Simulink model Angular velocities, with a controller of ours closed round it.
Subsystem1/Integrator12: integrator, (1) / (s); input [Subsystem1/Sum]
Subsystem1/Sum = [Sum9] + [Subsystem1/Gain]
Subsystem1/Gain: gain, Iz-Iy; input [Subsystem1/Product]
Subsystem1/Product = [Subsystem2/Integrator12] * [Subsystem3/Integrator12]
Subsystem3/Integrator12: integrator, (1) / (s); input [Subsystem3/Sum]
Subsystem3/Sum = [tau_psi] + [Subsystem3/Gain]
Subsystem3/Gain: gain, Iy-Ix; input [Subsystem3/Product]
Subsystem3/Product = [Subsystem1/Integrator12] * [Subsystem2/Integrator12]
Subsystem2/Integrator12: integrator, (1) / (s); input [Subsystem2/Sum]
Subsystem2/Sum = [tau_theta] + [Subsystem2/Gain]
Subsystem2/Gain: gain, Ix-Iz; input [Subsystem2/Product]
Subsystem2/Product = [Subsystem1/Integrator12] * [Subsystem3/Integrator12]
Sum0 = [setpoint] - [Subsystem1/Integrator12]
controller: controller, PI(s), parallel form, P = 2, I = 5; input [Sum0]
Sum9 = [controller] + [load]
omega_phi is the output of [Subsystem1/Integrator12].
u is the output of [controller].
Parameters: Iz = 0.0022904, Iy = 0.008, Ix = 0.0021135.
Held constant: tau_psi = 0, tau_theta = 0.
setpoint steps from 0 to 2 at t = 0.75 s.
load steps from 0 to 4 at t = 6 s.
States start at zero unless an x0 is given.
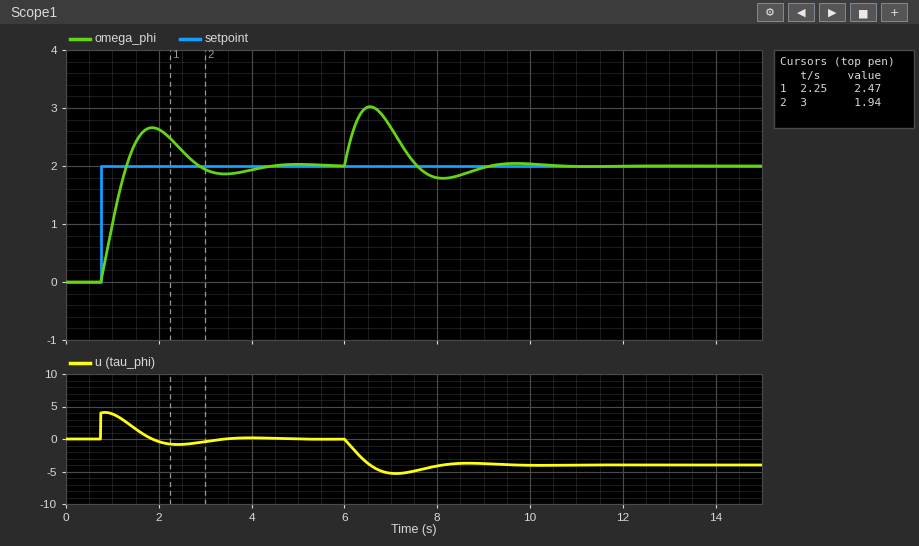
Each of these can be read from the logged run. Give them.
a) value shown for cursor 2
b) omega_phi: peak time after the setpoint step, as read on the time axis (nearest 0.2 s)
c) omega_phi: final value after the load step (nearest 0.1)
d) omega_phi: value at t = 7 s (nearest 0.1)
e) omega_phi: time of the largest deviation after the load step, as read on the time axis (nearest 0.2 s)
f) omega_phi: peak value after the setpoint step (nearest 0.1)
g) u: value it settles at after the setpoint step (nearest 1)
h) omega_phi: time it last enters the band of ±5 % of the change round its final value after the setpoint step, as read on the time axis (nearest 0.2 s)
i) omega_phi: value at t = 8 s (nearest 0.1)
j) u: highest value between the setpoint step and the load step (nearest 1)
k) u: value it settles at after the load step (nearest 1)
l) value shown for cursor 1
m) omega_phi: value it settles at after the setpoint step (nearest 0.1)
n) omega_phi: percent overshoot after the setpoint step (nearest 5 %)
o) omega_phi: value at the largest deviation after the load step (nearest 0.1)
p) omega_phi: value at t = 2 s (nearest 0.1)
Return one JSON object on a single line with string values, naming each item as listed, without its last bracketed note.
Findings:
{"value shown for cursor 2": "1.94", "omega_phi: peak time after the setpoint step, as read on the time axis": "1.8 s", "omega_phi: final value after the load step": "2.0", "omega_phi: value at t = 7 s": "2.7", "omega_phi: time of the largest deviation after the load step, as read on the time axis": "6.6 s", "omega_phi: peak value after the setpoint step": "2.7", "u: value it settles at after the setpoint step": "0", "omega_phi: time it last enters the band of ±5 % of the change round its final value after the setpoint step, as read on the time axis": "3.8 s", "omega_phi: value at t = 8 s": "1.8", "u: highest value between the setpoint step and the load step": "4", "u: value it settles at after the load step": "-4", "value shown for cursor 1": "2.47", "omega_phi: value it settles at after the setpoint step": "2.0", "omega_phi: percent overshoot after the setpoint step": "35 %", "omega_phi: value at the largest deviation after the load step": "3.0", "omega_phi: value at t = 2 s": "2.6"}
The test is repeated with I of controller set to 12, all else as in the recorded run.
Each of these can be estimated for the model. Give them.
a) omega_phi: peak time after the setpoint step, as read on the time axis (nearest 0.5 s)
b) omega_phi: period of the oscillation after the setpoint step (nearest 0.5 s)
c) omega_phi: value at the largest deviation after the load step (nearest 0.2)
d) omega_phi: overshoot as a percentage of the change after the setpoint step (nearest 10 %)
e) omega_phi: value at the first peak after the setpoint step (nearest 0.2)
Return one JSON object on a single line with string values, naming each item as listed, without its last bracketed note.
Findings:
{"omega_phi: peak time after the setpoint step, as read on the time axis": "1.5 s", "omega_phi: period of the oscillation after the setpoint step": "2.0 s", "omega_phi: value at the largest deviation after the load step": "2.8", "omega_phi: overshoot as a percentage of the change after the setpoint step": "50 %", "omega_phi: value at the first peak after the setpoint step": "3.0"}
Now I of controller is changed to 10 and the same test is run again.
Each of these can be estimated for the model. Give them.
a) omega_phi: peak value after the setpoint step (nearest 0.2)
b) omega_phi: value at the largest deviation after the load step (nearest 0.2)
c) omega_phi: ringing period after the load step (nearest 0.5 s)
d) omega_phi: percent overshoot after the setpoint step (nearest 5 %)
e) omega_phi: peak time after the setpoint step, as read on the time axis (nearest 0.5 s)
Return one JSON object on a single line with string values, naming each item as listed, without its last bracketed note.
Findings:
{"omega_phi: peak value after the setpoint step": "2.8", "omega_phi: value at the largest deviation after the load step": "2.8", "omega_phi: ringing period after the load step": "2.0 s", "omega_phi: percent overshoot after the setpoint step": "45 %", "omega_phi: peak time after the setpoint step, as read on the time axis": "1.5 s"}
